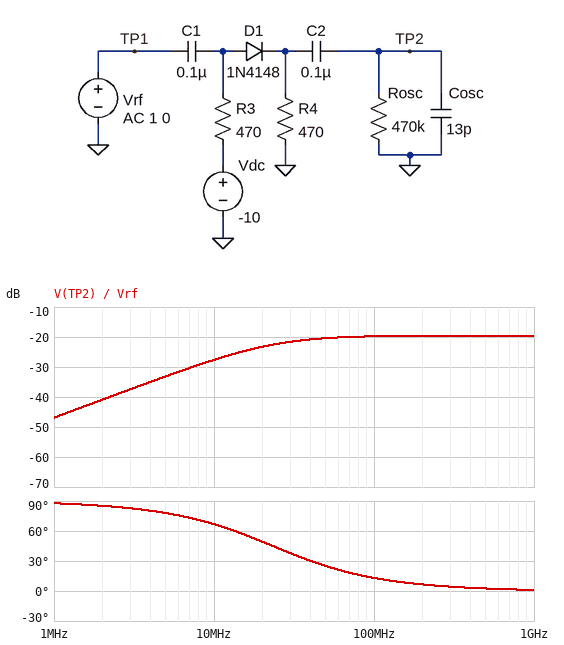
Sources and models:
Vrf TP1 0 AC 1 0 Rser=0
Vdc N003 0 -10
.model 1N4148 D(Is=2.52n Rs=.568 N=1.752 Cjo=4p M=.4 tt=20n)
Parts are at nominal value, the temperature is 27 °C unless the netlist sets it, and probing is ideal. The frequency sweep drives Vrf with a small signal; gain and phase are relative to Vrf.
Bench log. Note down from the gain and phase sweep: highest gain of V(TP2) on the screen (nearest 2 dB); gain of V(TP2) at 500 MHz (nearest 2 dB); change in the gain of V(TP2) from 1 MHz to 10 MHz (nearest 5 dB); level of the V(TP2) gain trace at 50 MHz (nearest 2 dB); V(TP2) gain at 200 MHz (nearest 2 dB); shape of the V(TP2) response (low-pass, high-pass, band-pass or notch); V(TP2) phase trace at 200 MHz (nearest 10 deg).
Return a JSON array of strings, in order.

["-20 dB", "-20 dB", "20 dB", "-20 dB", "-20 dB", "high-pass", "10 deg"]
